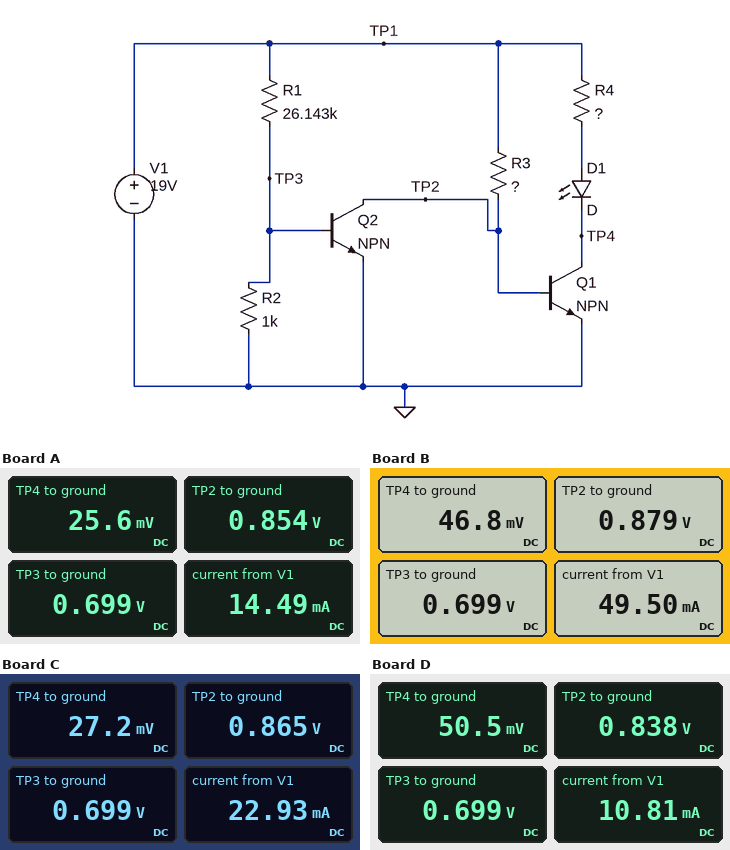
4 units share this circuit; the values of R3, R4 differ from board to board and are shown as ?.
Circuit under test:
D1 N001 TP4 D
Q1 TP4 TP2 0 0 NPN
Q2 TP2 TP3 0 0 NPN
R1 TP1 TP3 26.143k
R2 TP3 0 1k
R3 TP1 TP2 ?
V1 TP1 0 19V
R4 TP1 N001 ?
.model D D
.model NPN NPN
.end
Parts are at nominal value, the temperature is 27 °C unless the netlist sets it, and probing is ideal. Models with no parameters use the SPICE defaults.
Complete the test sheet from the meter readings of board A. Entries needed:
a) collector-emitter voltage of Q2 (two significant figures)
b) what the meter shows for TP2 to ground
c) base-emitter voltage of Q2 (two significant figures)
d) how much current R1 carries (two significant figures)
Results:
850 mV
0.854 V
700 mV
700 µA
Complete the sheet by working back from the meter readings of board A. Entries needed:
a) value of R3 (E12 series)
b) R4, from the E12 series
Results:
2.2 kΩ
3.3 kΩ
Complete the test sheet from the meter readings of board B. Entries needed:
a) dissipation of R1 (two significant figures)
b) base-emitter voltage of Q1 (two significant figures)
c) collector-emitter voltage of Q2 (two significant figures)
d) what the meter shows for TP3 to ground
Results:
13 mW
880 mV
880 mV
0.699 V
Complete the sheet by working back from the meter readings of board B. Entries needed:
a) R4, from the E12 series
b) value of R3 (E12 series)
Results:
470 Ω
1.8 kΩ
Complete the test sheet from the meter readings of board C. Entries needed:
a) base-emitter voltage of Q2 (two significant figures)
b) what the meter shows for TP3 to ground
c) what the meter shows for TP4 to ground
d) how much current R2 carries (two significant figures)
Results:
700 mV
0.699 V
27.2 mV
700 µA
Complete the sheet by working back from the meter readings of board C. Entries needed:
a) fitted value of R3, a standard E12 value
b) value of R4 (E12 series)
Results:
1.5 kΩ
1.8 kΩ
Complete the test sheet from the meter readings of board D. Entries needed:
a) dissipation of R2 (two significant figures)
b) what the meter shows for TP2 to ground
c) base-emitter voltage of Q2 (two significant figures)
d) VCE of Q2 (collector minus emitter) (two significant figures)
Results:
490 µW
0.838 V
700 mV
840 mV
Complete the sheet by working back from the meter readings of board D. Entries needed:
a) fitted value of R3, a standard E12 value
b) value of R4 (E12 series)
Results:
10 kΩ
2.2 kΩ
